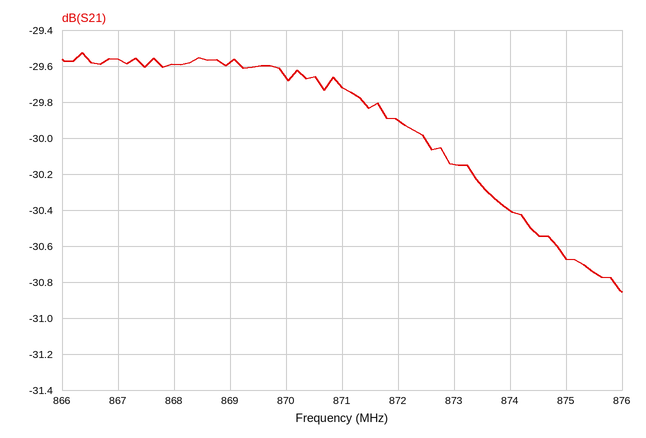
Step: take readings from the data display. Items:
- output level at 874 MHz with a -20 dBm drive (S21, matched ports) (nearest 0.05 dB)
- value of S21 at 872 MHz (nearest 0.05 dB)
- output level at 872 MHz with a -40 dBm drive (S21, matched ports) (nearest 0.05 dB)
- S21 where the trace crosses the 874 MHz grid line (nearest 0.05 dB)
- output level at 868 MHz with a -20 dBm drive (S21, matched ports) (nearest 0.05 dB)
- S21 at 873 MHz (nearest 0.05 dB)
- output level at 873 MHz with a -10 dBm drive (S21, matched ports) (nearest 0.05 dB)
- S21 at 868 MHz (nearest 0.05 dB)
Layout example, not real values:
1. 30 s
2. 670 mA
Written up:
1. -50.40 dBm
2. -29.90 dB
3. -69.90 dBm
4. -30.40 dB
5. -49.60 dBm
6. -30.15 dB
7. -40.15 dBm
8. -29.60 dB
